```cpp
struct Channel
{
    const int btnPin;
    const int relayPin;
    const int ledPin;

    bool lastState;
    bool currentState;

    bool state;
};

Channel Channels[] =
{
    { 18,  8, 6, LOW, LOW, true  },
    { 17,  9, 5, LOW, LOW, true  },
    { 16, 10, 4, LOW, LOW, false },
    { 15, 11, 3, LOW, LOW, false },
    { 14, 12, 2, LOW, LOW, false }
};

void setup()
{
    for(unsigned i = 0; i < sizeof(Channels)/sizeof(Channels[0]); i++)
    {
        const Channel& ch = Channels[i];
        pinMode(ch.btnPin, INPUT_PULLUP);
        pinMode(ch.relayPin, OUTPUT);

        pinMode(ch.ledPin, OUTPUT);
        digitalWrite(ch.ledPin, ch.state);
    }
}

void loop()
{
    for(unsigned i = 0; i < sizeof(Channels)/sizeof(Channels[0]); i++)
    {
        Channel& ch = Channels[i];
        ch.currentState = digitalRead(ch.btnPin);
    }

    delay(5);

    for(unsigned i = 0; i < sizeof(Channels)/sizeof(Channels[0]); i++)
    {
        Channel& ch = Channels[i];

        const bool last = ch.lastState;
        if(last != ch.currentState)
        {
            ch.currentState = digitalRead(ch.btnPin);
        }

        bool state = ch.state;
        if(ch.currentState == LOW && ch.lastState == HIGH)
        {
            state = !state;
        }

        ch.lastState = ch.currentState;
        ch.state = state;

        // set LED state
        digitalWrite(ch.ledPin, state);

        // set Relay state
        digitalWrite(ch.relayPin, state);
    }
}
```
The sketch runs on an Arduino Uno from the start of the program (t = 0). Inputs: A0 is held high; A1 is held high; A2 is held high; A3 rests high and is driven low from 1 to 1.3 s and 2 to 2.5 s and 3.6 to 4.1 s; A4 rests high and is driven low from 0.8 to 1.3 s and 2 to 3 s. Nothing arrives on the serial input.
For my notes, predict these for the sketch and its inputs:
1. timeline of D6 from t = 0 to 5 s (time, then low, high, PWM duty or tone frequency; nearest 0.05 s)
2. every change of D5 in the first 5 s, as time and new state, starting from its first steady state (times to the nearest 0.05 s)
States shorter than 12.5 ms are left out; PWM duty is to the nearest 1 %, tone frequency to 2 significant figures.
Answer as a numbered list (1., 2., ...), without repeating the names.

1. 0 s high; 0.8 s low; 2 s high
2. 0 s high; 1 s low; 2 s high; 3.6 s low
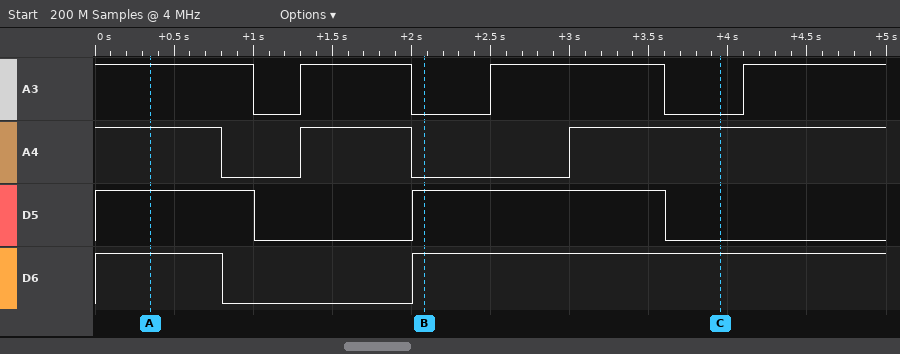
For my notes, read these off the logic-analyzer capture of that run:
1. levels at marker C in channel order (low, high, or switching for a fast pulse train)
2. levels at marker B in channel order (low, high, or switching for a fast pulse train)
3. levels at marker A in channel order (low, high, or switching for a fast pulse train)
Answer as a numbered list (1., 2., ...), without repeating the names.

1. A3 low, A4 high, D5 low, D6 high
2. A3 low, A4 low, D5 high, D6 high
3. A3 high, A4 high, D5 high, D6 high
